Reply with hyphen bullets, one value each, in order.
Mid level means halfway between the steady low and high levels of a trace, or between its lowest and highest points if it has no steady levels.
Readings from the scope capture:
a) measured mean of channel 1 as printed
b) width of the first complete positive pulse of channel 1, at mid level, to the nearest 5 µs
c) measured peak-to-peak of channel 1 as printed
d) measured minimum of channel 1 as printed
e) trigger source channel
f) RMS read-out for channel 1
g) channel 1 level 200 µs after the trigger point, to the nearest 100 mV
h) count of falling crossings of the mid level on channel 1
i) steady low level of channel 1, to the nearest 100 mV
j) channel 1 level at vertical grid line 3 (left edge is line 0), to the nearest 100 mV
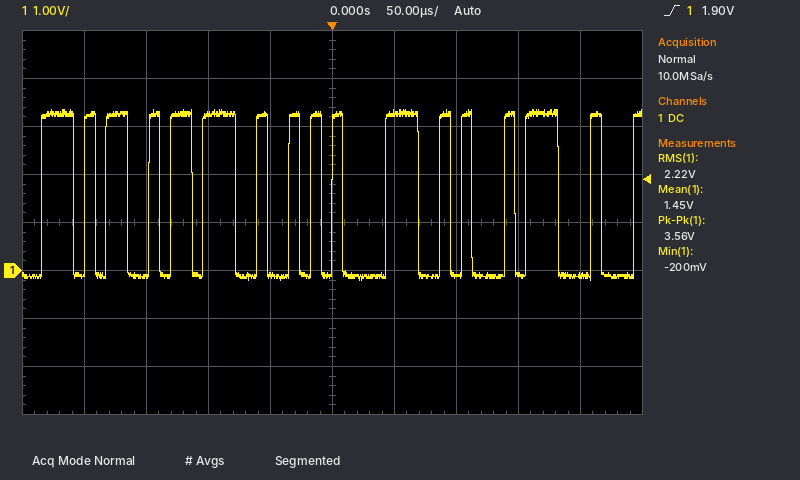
- 1.45 V
- 25 µs
- 3.56 V
- -200 mV
- channel 1
- 2.22 V
- -100 mV
- 16
- -100 mV
- 3.2 V
